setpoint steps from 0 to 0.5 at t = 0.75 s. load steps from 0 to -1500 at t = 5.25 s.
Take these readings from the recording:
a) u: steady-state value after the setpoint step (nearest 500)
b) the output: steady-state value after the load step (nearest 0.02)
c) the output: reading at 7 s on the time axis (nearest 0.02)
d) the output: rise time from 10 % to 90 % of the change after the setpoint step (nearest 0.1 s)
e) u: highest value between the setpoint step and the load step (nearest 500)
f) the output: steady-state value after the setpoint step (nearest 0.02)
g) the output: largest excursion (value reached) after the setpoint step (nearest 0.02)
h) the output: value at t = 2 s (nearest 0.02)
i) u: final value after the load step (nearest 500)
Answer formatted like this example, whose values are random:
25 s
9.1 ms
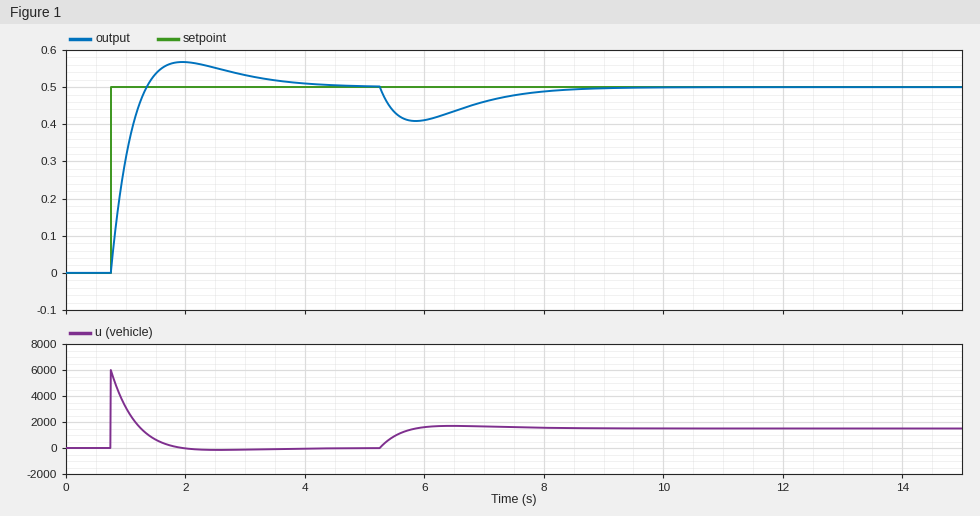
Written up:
0
0.50
0.46
0.4 s
6000
0.50
0.56
0.56
1500
